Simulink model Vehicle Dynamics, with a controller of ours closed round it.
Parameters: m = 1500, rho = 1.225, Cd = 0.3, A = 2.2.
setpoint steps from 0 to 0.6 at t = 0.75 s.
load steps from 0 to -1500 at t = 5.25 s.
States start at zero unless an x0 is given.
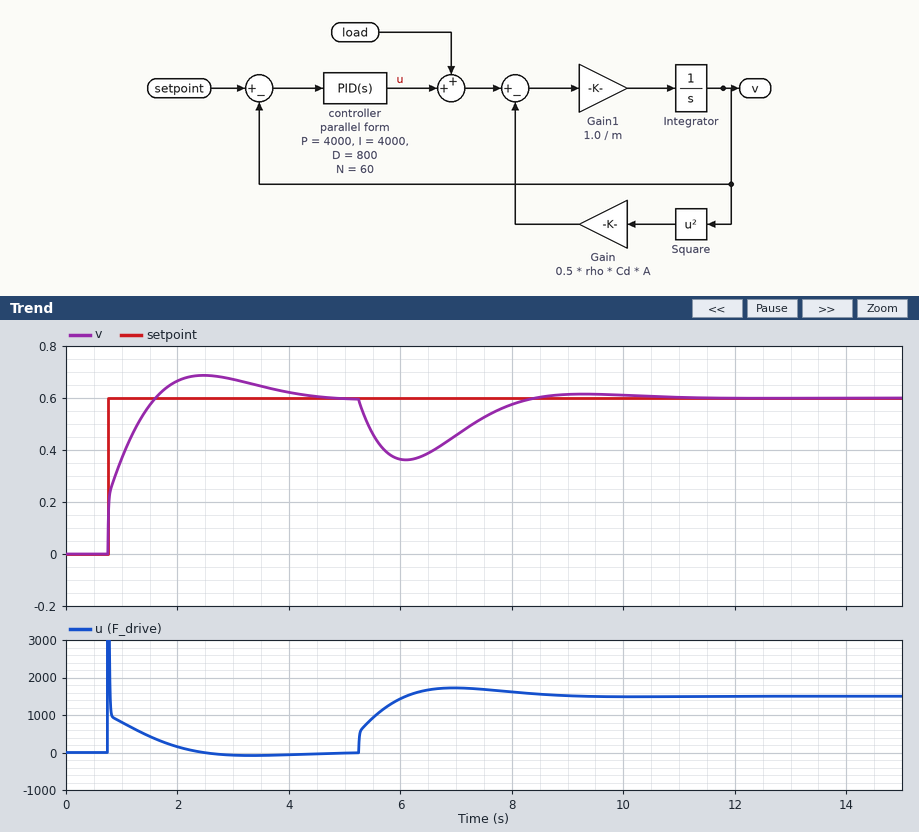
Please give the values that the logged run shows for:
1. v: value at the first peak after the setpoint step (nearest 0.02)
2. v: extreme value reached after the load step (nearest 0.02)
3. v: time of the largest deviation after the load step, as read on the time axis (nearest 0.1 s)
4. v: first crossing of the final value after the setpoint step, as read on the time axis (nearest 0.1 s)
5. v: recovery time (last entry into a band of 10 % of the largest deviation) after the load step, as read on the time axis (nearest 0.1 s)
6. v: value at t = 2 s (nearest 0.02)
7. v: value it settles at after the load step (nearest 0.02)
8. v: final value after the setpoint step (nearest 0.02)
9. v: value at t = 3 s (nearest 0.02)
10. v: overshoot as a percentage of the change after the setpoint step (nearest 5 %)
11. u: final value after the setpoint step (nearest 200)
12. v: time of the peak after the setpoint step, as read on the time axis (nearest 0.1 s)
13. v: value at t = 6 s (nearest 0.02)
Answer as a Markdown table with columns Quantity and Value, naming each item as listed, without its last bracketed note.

| Quantity | Value |
|---|---|
| v: value at the first peak after the setpoint step | 0.68 |
| v: extreme value reached after the load step | 0.36 |
| v: time of the largest deviation after the load step, as read on the time axis | 6.1 s |
| v: first crossing of the final value after the setpoint step, as read on the time axis | 1.6 s |
| v: recovery time (last entry into a band of 10 % of the largest deviation) after the load step, as read on the time axis | 8.0 s |
| v: value at t = 2 s | 0.66 |
| v: value it settles at after the load step | 0.60 |
| v: final value after the setpoint step | 0.60 |
| v: value at t = 3 s | 0.68 |
| v: overshoot as a percentage of the change after the setpoint step | 15 % |
| u: final value after the setpoint step | 0 |
| v: time of the peak after the setpoint step, as read on the time axis | 2.5 s |
| v: value at t = 6 s | 0.36 |
